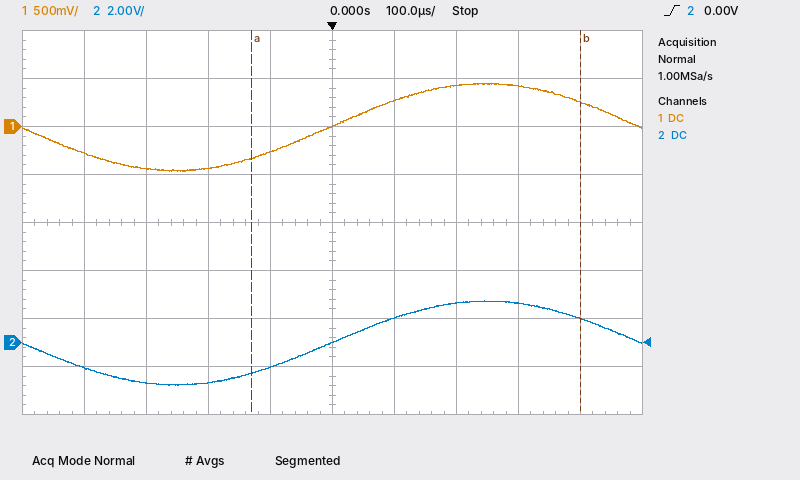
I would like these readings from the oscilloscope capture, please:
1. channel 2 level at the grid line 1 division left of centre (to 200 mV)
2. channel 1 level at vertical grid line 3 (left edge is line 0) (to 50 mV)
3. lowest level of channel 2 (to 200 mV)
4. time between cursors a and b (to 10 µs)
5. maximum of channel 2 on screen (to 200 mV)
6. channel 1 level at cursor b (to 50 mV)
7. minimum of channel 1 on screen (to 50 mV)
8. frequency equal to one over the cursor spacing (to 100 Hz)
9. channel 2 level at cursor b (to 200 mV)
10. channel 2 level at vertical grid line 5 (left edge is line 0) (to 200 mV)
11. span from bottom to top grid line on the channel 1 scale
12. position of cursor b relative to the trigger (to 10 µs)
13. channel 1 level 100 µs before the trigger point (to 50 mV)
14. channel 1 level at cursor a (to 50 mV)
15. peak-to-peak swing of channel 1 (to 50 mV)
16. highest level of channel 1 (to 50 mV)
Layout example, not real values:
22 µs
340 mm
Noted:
-1.0 V
-450 mV
-1.8 V
530 µs
1.8 V
250 mV
-450 mV
1.9 kHz
1.0 V
0.0 V
4 V
+400 µs
-250 mV
-350 mV
900 mV
450 mV
